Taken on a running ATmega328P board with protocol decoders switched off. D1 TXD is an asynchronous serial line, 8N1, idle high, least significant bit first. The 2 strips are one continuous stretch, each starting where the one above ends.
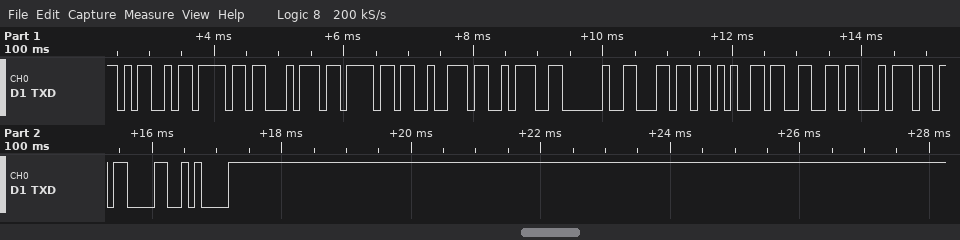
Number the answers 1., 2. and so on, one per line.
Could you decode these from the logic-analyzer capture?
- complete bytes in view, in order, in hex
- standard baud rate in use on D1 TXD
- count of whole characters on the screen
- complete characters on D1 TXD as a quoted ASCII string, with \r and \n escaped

1. 4D 6F 74 6F 72 3A 20 6C 65 66 74 0D 0A
2. 9600 baud
3. 13
4. "Motor: left\r\n"
